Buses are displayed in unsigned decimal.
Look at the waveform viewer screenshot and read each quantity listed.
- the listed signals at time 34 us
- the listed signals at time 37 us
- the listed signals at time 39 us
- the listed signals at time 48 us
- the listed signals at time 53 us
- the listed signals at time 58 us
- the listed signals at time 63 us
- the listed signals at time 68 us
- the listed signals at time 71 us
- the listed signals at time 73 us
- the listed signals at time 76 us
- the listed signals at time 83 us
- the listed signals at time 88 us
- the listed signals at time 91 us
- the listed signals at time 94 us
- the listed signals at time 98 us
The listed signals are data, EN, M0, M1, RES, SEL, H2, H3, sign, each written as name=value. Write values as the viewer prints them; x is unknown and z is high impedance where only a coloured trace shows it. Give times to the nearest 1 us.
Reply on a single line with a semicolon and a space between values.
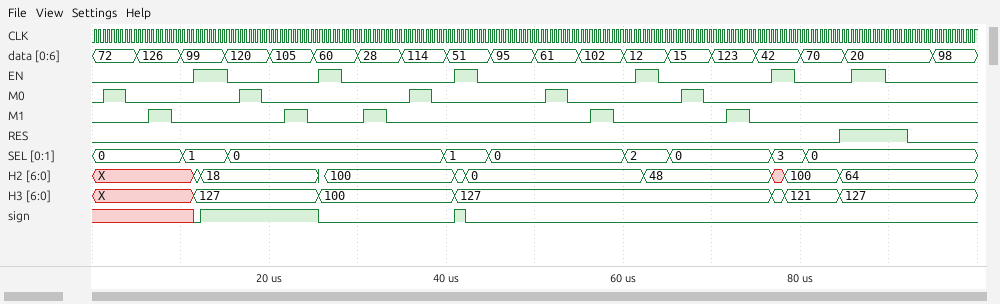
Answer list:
data=28, EN=0, M0=0, M1=0, RES=0, SEL=0, H2=100, H3=100, sign=0; data=114, EN=0, M0=1, M1=0, RES=0, SEL=0, H2=100, H3=100, sign=0; data=114, EN=0, M0=0, M1=0, RES=0, SEL=0, H2=100, H3=100, sign=0; data=95, EN=0, M0=0, M1=0, RES=0, SEL=0, H2=0, H3=127, sign=0; data=61, EN=0, M0=1, M1=0, RES=0, SEL=0, H2=0, H3=127, sign=0; data=102, EN=0, M0=0, M1=1, RES=0, SEL=0, H2=0, H3=127, sign=0; data=12, EN=1, M0=0, M1=0, RES=0, SEL=2, H2=48, H3=127, sign=0; data=15, EN=0, M0=1, M1=0, RES=0, SEL=0, H2=48, H3=127, sign=0; data=123, EN=0, M0=0, M1=0, RES=0, SEL=0, H2=48, H3=127, sign=0; data=123, EN=0, M0=0, M1=1, RES=0, SEL=0, H2=48, H3=127, sign=0; data=42, EN=0, M0=0, M1=0, RES=0, SEL=0, H2=48, H3=127, sign=0; data=70, EN=0, M0=0, M1=0, RES=0, SEL=0, H2=100, H3=121, sign=0; data=20, EN=1, M0=0, M1=0, RES=1, SEL=0, H2=64, H3=127, sign=0; data=20, EN=0, M0=0, M1=0, RES=1, SEL=0, H2=64, H3=127, sign=0; data=20, EN=0, M0=0, M1=0, RES=0, SEL=0, H2=64, H3=127, sign=0; data=98, EN=0, M0=0, M1=0, RES=0, SEL=0, H2=64, H3=127, sign=0
